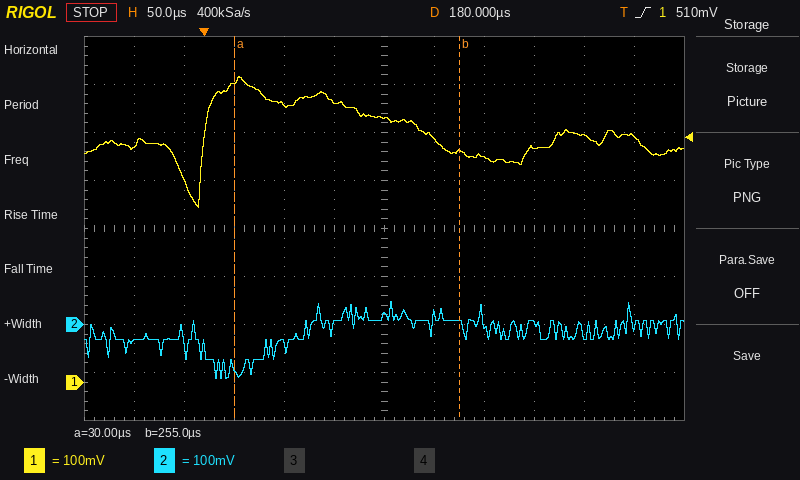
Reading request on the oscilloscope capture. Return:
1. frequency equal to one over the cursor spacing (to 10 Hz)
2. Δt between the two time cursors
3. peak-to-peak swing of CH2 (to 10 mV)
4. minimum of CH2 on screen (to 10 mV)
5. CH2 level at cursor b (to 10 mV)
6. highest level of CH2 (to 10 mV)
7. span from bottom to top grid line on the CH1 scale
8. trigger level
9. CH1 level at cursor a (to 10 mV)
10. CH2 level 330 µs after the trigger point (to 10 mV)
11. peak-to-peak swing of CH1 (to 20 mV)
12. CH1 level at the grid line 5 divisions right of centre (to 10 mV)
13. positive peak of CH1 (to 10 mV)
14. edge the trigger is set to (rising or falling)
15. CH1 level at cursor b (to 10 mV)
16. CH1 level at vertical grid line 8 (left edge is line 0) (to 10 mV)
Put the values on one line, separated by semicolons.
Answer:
4.44 kHz; 225 µs; 160 mV; -110 mV; 0 mV; 50 mV; 800 mV; 510 mV; 630 mV; 0 mV; 280 mV; 510 mV; 640 mV; rising; 480 mV; 470 mV
